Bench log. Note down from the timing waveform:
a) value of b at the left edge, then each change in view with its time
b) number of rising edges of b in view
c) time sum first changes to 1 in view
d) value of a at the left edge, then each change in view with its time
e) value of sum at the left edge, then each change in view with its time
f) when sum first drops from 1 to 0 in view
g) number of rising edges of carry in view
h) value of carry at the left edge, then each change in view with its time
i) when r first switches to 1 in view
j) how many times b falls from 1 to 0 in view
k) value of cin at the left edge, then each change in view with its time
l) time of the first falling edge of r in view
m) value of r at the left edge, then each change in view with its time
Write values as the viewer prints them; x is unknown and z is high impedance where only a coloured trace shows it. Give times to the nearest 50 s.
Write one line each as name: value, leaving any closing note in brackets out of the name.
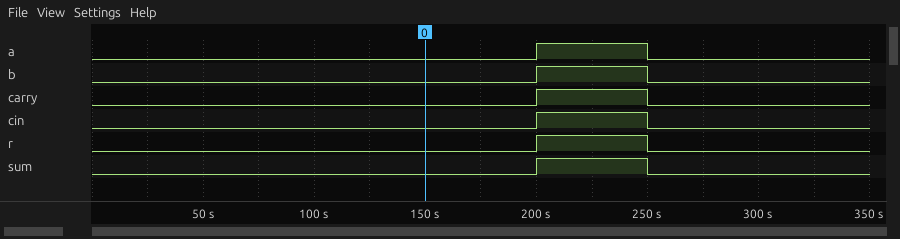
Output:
value of b at the left edge, then each change in view with its time: 0, 1 at 200 s, 0 at 250 s
number of rising edges of b in view: 1
time sum first changes to 1 in view: 200 s
value of a at the left edge, then each change in view with its time: 0, 1 at 200 s, 0 at 250 s
value of sum at the left edge, then each change in view with its time: 0, 1 at 200 s, 0 at 250 s
when sum first drops from 1 to 0 in view: 250 s
number of rising edges of carry in view: 1
value of carry at the left edge, then each change in view with its time: 0, 1 at 200 s, 0 at 250 s
when r first switches to 1 in view: 200 s
how many times b falls from 1 to 0 in view: 1
value of cin at the left edge, then each change in view with its time: 0, 1 at 200 s, 0 at 250 s
time of the first falling edge of r in view: 250 s
value of r at the left edge, then each change in view with its time: 0, 1 at 200 s, 0 at 250 s
